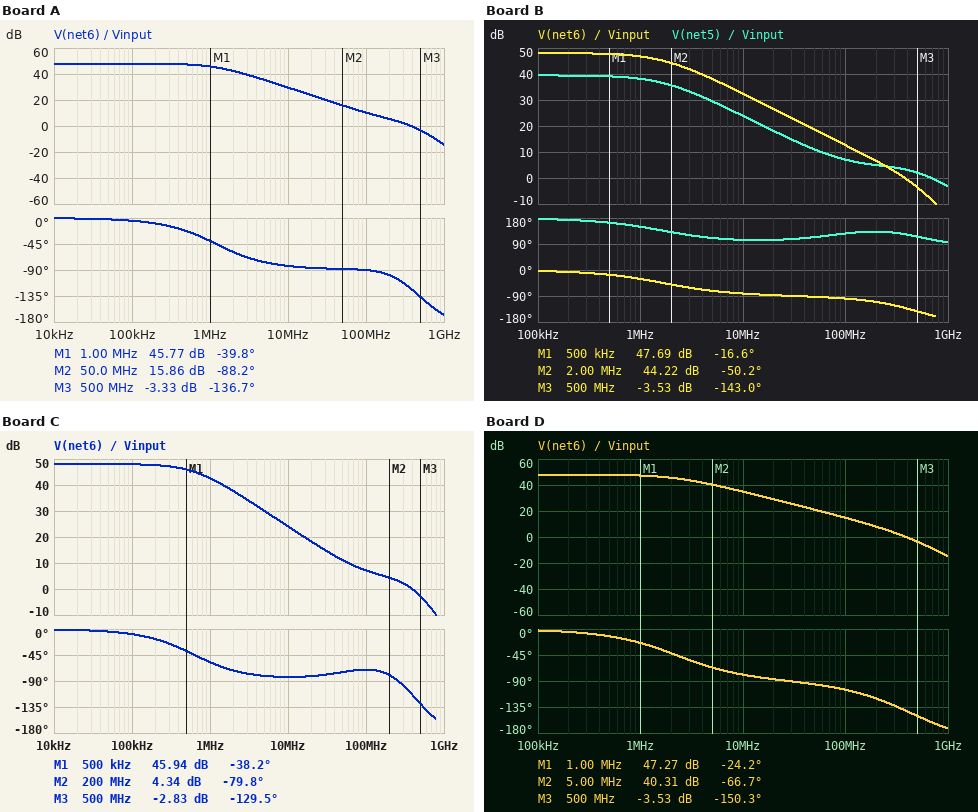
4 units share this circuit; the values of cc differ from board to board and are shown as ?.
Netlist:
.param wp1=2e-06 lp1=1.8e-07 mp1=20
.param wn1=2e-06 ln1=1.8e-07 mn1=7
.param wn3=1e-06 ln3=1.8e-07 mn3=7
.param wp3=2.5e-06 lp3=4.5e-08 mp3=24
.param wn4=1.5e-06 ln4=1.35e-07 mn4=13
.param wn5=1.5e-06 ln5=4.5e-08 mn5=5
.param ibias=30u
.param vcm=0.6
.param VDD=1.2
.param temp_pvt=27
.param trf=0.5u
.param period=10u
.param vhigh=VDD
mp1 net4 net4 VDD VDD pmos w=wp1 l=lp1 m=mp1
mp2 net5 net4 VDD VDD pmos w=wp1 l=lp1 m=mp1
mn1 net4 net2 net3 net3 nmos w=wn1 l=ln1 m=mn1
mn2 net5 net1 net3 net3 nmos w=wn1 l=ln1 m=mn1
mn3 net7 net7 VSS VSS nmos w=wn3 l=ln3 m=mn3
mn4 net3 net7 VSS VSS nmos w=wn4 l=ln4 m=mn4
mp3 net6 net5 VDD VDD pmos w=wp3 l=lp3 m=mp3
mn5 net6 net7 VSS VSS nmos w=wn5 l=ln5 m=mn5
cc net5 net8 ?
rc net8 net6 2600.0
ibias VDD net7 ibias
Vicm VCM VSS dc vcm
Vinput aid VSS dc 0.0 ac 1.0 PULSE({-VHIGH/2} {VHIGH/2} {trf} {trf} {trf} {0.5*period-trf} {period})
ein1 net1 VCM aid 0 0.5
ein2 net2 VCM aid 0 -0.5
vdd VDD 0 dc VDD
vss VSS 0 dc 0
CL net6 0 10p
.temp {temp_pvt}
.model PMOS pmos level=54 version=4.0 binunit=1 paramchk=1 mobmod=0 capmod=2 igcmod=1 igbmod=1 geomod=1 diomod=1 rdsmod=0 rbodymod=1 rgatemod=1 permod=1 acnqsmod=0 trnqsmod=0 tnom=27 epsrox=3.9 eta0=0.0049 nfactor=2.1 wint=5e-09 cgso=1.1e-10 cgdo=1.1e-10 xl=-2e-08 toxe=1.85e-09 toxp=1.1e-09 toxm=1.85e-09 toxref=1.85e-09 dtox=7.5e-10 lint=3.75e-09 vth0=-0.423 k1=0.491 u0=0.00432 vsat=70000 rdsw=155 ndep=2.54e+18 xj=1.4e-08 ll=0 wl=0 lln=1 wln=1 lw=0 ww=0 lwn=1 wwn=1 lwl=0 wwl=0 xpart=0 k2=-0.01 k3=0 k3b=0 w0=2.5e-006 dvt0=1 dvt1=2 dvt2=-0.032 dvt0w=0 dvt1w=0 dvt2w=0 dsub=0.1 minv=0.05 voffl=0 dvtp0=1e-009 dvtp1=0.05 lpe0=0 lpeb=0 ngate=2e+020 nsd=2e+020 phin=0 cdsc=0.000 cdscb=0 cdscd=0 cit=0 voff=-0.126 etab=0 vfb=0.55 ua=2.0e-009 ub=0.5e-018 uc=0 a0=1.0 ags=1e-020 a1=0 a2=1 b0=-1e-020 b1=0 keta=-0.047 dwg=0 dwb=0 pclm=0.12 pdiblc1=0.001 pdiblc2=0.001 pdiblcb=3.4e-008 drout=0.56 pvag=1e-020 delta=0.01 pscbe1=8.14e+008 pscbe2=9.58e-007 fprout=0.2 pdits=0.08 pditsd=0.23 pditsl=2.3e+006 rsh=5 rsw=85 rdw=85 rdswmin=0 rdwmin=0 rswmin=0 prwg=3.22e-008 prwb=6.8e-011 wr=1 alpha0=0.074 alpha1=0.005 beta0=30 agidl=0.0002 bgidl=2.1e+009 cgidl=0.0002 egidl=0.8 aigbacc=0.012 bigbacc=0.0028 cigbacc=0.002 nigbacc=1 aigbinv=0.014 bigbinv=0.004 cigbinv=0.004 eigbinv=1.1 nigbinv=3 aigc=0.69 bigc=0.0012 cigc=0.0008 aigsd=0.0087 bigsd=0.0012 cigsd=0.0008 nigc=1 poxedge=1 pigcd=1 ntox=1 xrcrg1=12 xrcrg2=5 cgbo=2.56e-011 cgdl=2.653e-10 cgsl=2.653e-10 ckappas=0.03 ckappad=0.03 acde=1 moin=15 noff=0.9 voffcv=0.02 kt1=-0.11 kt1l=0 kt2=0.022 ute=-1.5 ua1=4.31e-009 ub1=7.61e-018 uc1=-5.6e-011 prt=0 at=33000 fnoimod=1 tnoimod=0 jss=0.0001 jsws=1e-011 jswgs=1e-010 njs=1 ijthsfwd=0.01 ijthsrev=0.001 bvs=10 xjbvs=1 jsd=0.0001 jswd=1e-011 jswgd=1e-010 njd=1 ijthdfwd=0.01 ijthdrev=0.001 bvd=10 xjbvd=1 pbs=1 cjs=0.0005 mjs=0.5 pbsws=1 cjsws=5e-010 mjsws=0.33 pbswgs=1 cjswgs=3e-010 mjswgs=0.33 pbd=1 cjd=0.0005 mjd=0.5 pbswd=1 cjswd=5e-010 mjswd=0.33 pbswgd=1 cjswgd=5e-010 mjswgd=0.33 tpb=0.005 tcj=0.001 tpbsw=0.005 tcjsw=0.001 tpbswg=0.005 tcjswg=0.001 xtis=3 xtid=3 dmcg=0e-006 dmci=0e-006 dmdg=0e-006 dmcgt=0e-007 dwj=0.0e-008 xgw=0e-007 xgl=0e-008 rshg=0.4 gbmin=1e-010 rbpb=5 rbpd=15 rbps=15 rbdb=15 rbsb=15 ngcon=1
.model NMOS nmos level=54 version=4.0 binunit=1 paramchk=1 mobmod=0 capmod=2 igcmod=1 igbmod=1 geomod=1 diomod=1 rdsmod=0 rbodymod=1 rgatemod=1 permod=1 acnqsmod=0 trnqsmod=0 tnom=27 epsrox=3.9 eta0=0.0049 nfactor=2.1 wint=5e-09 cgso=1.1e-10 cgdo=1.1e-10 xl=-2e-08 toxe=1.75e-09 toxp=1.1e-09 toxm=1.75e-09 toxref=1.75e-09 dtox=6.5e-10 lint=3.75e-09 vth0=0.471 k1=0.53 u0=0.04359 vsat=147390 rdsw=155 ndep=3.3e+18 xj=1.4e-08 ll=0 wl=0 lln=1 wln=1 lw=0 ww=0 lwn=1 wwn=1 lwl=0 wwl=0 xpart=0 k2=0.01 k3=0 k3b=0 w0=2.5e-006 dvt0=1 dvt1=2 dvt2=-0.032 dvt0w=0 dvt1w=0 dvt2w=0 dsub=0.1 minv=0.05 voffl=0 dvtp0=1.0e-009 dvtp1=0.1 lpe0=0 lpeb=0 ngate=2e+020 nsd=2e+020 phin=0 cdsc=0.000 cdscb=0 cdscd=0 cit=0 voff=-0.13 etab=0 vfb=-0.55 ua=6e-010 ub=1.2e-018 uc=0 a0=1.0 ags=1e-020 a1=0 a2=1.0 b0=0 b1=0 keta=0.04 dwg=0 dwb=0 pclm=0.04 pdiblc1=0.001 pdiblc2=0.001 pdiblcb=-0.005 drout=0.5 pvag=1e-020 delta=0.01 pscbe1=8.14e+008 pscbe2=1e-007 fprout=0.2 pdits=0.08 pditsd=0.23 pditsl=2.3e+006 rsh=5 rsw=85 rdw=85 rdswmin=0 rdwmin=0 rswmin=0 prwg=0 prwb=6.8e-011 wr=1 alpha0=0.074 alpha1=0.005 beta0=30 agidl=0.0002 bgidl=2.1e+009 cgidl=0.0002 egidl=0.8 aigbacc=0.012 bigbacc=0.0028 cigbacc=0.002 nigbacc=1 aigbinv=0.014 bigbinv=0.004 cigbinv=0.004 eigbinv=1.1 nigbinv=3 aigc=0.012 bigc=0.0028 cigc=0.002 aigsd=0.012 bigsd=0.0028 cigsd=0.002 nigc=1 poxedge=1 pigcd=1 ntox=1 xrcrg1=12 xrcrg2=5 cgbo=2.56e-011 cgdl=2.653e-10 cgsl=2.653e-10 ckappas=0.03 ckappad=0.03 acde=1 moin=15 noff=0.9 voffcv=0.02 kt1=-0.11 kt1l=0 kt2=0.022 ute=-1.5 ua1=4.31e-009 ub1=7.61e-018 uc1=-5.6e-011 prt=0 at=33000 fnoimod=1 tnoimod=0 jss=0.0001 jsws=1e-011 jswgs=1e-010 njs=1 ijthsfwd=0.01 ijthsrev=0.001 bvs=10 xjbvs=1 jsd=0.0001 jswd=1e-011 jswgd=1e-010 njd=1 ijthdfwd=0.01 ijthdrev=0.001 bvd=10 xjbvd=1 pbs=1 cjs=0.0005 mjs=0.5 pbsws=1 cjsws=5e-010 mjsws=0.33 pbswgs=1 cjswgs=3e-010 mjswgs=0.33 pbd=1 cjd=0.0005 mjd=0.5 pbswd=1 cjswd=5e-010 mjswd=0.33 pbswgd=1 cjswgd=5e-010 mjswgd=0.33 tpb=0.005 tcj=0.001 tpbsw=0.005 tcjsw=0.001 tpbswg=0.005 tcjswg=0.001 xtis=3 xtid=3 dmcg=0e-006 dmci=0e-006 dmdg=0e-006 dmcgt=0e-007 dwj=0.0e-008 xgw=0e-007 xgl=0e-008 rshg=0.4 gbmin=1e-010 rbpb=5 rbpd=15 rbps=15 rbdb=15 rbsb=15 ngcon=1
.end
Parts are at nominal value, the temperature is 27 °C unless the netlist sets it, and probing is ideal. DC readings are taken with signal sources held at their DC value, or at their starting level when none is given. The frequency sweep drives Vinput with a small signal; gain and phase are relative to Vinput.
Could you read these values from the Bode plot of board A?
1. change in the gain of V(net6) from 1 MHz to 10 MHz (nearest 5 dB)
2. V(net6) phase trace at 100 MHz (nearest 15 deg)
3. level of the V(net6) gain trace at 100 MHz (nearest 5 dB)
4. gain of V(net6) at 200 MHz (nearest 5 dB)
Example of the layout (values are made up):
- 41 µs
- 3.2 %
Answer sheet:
- -15 dB
- -90 deg
- 10 dB
- 5 dB
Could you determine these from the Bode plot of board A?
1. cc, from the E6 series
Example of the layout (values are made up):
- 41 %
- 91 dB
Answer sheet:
- 330 fF
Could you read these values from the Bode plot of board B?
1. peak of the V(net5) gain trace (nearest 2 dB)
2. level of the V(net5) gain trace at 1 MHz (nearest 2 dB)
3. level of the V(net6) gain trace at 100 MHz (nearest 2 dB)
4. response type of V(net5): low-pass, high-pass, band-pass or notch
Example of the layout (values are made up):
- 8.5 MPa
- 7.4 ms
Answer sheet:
- 40 dB
- 38 dB
- 12 dB
- low-pass
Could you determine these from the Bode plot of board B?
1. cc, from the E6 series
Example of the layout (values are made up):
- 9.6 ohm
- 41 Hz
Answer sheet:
- 220 fF
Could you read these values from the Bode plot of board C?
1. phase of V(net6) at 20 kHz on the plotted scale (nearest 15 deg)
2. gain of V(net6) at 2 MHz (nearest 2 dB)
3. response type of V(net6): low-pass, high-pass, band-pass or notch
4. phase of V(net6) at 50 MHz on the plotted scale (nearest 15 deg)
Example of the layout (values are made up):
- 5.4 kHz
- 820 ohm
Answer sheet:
- 0 deg
- 38 dB
- low-pass
- -75 deg
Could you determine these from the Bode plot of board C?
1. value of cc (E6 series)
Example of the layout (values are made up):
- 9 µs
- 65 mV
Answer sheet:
- 680 fF
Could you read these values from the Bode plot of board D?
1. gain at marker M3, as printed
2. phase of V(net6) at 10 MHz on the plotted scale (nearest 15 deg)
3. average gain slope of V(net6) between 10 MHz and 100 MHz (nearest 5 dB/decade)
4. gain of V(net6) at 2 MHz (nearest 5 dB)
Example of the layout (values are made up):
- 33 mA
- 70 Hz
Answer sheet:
- -3.53 dB
- -75 deg
- -20 dB/decade
- 45 dB
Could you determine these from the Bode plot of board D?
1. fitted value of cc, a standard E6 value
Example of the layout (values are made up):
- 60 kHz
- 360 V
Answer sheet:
- 150 fF
